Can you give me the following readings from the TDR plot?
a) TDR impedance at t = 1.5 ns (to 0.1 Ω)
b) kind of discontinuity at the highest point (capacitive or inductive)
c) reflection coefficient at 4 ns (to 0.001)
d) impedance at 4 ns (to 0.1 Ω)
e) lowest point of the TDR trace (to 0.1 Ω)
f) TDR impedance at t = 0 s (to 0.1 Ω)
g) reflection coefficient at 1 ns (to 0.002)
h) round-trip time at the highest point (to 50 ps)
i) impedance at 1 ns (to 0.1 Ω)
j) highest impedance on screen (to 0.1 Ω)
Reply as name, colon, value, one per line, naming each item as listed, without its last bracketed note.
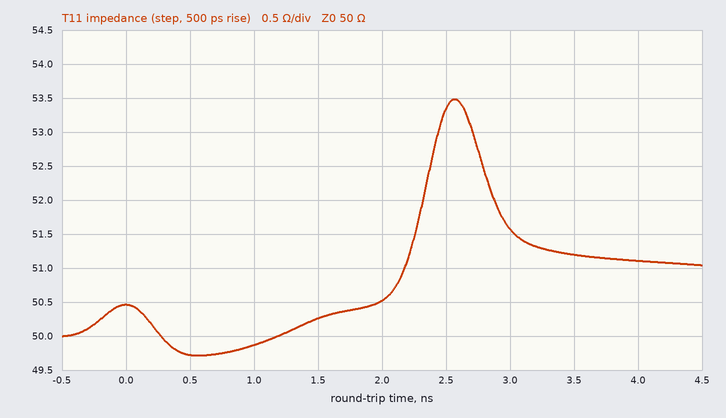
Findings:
TDR impedance at t = 1.5 ns: 50.3 Ω
kind of discontinuity at the highest point: inductive
reflection coefficient at 4 ns: +0.011
impedance at 4 ns: 51.1 Ω
lowest point of the TDR trace: 49.7 Ω
TDR impedance at t = 0 s: 50.5 Ω
reflection coefficient at 1 ns: -0.002
round-trip time at the highest point: 2.55 ns
impedance at 1 ns: 49.9 Ω
highest impedance on screen: 53.5 Ω
